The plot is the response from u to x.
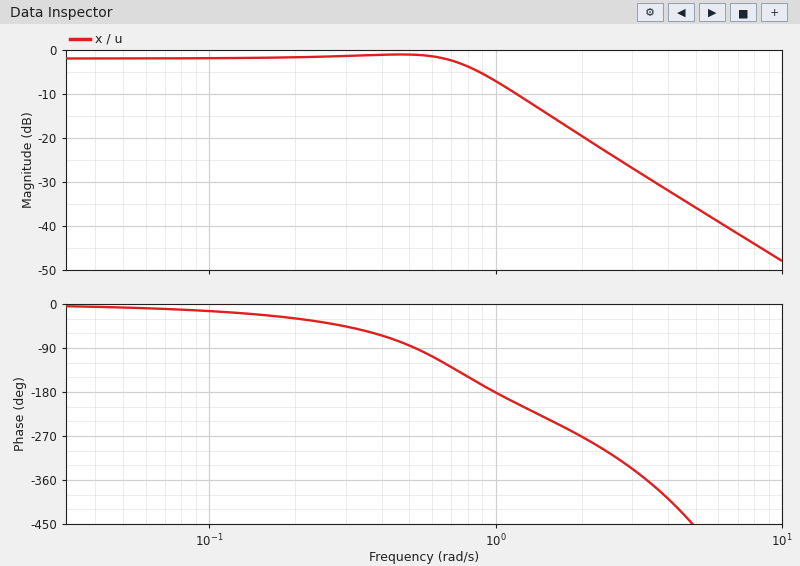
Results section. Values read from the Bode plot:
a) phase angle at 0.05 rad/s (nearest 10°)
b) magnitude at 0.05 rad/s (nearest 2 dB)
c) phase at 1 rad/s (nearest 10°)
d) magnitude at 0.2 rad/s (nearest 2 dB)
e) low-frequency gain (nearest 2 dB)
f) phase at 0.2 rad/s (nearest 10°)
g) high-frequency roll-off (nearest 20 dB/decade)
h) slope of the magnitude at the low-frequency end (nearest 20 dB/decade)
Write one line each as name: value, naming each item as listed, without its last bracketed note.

phase angle at 0.05 rad/s: -10°
magnitude at 0.05 rad/s: -2 dB
phase at 1 rad/s: -180°
magnitude at 0.2 rad/s: -2 dB
low-frequency gain: -2 dB
phase at 0.2 rad/s: -30°
high-frequency roll-off: -40 dB/decade
slope of the magnitude at the low-frequency end: 0 dB/decade
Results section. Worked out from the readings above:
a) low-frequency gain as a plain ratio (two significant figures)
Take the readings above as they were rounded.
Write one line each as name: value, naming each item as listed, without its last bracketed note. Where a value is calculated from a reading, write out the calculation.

low-frequency gain as a plain ratio: 10^(-2 / 20) = 0.79
